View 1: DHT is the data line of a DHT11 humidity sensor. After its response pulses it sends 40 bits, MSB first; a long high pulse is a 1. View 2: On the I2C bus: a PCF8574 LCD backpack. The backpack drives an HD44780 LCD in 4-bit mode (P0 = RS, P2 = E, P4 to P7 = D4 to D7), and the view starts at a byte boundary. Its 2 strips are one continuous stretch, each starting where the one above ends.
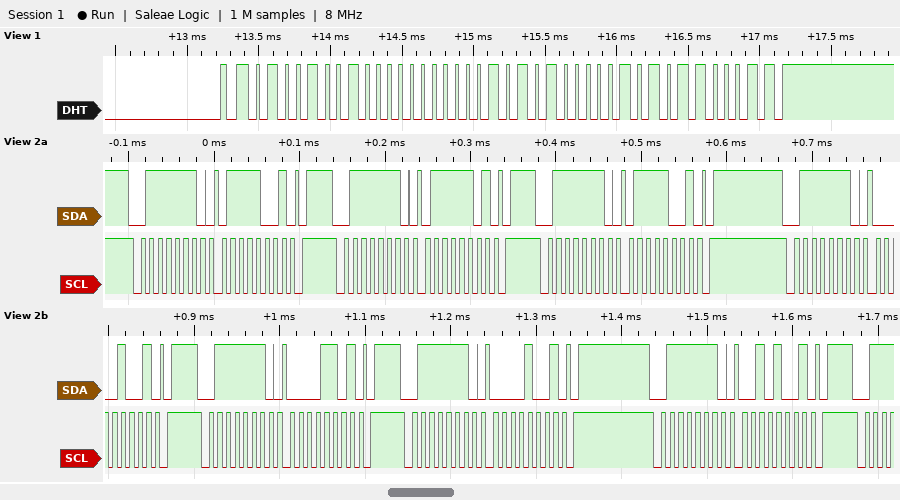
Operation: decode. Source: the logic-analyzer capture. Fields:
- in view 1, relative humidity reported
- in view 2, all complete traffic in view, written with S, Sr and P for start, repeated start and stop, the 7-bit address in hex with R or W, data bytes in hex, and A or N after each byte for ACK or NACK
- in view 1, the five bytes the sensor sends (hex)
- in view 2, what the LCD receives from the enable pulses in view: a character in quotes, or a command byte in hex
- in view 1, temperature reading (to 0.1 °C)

73 %
S 3FW A 79 A P S 3FW A 7D A P S 3FW A 79 A P S 3FW A 09 A P S 3FW A 0D A P S 3FW A 09 A P S 3FW A 29 A P
49 00 15 05 63
'p'
21.5 °C
